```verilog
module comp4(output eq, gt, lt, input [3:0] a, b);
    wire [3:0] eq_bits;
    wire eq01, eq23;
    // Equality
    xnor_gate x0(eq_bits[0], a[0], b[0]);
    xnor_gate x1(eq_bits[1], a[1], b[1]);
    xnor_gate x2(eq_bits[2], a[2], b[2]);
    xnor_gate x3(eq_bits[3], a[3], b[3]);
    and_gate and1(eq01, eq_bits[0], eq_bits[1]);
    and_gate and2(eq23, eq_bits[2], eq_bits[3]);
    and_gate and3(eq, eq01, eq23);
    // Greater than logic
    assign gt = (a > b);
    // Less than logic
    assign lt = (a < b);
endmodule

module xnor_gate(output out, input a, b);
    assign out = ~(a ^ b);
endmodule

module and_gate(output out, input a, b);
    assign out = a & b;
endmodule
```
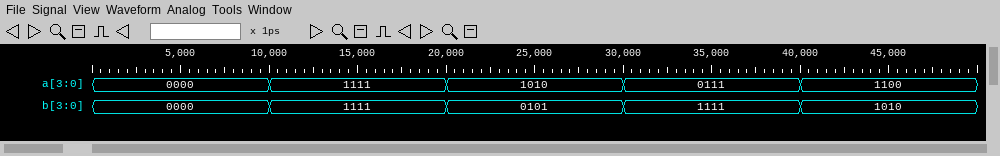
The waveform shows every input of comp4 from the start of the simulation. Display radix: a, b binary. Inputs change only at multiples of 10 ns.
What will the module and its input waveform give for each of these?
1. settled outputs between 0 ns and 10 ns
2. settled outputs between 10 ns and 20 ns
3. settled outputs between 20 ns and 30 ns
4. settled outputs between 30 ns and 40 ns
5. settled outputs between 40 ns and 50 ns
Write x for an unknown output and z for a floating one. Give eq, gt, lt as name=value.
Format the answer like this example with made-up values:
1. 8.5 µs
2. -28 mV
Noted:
1. eq=1, gt=0, lt=0
2. eq=1, gt=0, lt=0
3. eq=0, gt=1, lt=0
4. eq=0, gt=0, lt=1
5. eq=0, gt=1, lt=0
